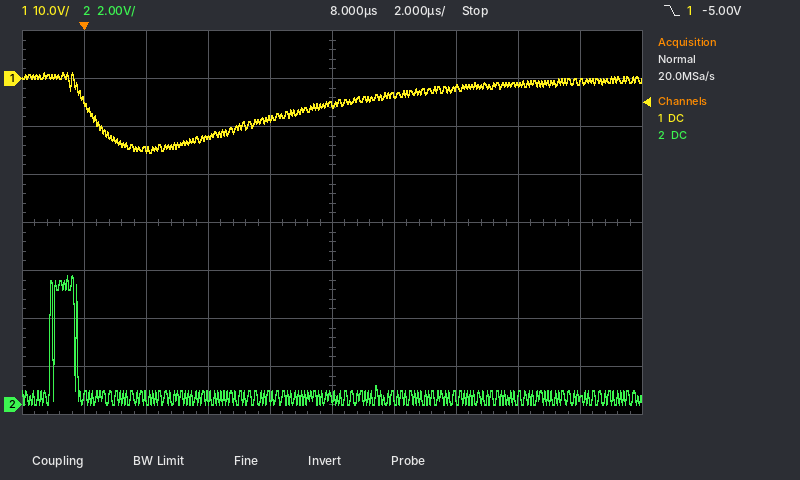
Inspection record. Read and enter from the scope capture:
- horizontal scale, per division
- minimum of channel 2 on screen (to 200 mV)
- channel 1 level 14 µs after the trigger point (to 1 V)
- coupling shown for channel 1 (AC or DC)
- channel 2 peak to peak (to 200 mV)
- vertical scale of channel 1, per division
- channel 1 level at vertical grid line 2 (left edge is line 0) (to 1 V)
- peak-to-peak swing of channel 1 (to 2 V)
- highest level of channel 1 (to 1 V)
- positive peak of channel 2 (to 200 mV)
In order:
2 µs
0.0 V
-1 V
DC
5.4 V
10 V
-15 V
16 V
1 V
5.4 V
